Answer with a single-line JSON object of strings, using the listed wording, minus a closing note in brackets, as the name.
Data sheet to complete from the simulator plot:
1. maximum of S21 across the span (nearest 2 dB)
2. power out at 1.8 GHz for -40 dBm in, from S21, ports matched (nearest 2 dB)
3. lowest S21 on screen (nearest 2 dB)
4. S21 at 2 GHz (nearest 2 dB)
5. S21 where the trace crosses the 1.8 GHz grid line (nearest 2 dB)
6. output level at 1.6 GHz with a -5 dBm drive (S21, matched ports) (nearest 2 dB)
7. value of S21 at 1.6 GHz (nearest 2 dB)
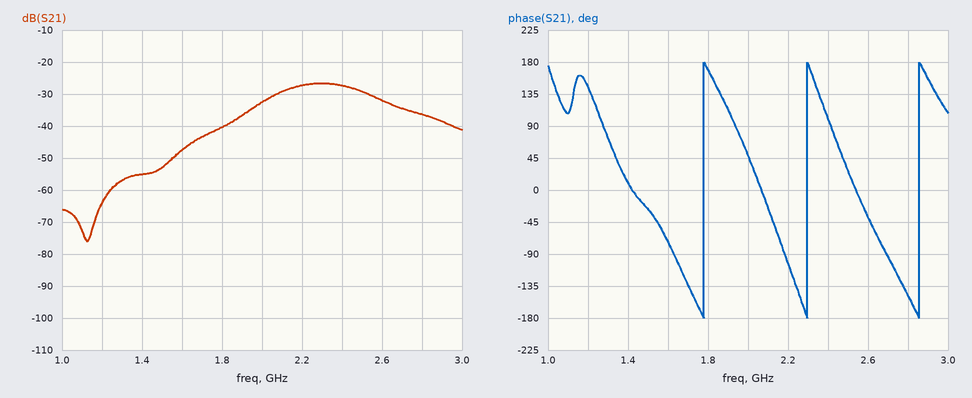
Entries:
{"maximum of S21 across the span": "-26 dB", "power out at 1.8 GHz for -40 dBm in, from S21, ports matched": "-80 dBm", "lowest S21 on screen": "-76 dB", "S21 at 2 GHz": "-32 dB", "S21 where the trace crosses the 1.8 GHz grid line": "-40 dB", "output level at 1.6 GHz with a -5 dBm drive (S21, matched ports)": "-52 dBm", "value of S21 at 1.6 GHz": "-48 dB"}
